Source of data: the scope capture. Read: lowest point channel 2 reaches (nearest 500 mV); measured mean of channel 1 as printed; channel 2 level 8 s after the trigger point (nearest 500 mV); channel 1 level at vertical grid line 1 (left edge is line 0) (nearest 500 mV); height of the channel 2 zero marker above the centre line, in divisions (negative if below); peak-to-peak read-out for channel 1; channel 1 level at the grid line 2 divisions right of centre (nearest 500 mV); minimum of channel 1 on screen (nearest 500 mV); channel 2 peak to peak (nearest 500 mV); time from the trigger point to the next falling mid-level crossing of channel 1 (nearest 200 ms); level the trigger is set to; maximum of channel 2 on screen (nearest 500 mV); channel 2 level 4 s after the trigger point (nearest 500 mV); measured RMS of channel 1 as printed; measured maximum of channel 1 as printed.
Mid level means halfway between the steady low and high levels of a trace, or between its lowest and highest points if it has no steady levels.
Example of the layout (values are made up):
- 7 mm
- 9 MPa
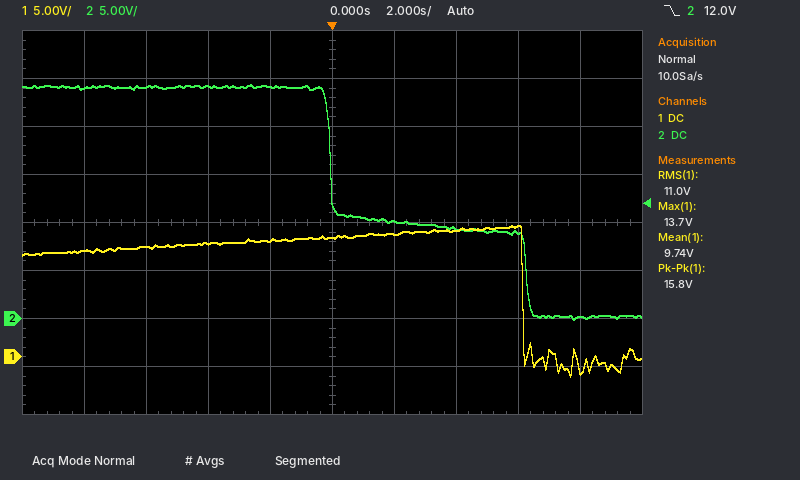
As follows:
- 0.0 V
- 9.74 V
- 0.0 V
- 11.0 V
- -2.0 div
- 15.8 V
- 13.0 V
- -2.0 V
- 24.5 V
- 6.2 s
- 12.0 V
- 24.5 V
- 9.5 V
- 11.0 V
- 13.7 V
